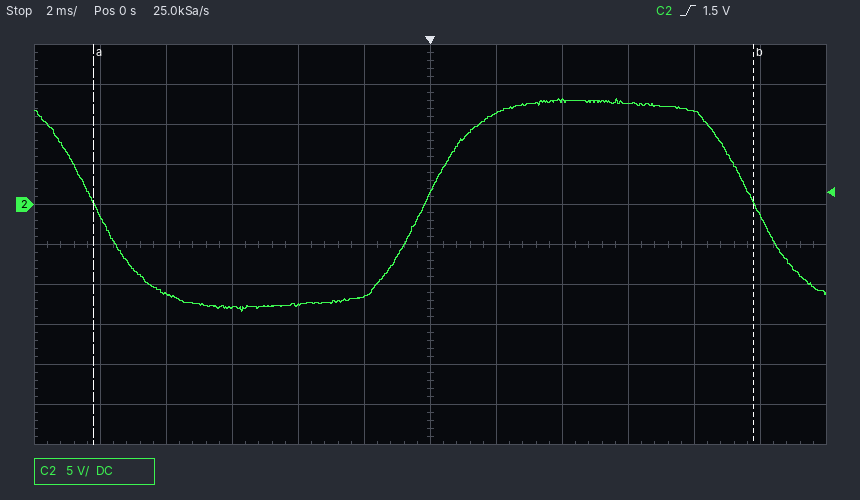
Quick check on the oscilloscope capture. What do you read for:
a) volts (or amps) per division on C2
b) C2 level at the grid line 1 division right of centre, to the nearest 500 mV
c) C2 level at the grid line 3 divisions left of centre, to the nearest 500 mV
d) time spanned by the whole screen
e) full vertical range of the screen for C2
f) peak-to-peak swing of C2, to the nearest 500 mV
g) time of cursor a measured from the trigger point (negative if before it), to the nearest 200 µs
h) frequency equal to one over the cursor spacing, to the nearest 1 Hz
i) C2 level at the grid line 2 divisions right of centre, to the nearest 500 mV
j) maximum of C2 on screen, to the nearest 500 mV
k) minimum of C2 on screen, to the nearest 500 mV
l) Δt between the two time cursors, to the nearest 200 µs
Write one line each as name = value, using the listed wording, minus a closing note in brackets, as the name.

volts (or amps) per division on C2 = 5 V
C2 level at the grid line 1 division right of centre, to the nearest 500 mV = 11.5 V
C2 level at the grid line 3 divisions left of centre, to the nearest 500 mV = -13.0 V
time spanned by the whole screen = 24 ms
full vertical range of the screen for C2 = 50 V
peak-to-peak swing of C2, to the nearest 500 mV = 26.5 V
time of cursor a measured from the trigger point (negative if before it), to the nearest 200 µs = -10.2 ms
frequency equal to one over the cursor spacing, to the nearest 1 Hz = 50 Hz
C2 level at the grid line 2 divisions right of centre, to the nearest 500 mV = 13.0 V
maximum of C2 on screen, to the nearest 500 mV = 13.0 V
minimum of C2 on screen, to the nearest 500 mV = -13.5 V
Δt between the two time cursors, to the nearest 200 µs = 20.0 ms
